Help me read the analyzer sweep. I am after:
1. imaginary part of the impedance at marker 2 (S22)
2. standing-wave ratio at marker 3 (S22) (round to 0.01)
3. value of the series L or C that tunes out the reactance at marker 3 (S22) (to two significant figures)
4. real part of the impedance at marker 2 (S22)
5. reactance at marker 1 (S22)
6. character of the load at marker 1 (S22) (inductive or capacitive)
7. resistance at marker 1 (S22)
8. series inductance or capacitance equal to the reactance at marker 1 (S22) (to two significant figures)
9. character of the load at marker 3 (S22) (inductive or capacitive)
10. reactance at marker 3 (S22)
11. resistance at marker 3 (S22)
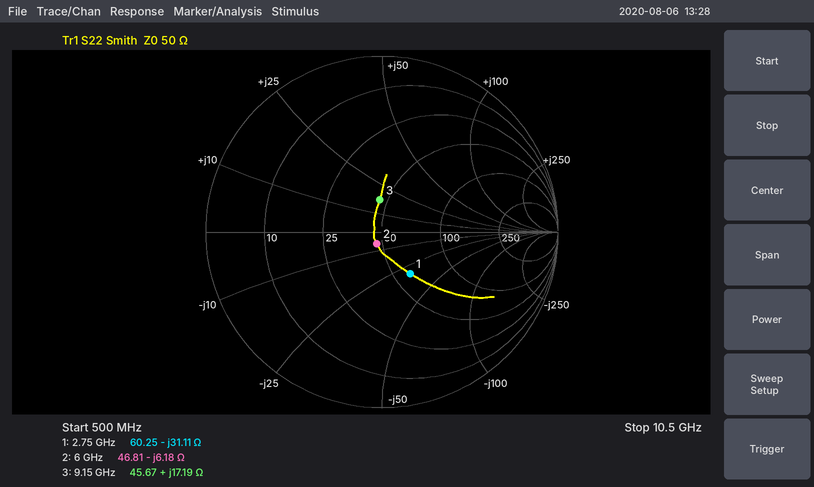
-6.18 Ω
1.45
1.0 pF
46.81 Ω
-31.11 Ω
capacitive
60.25 Ω
1.9 pF
inductive
+17.19 Ω
45.67 Ω
